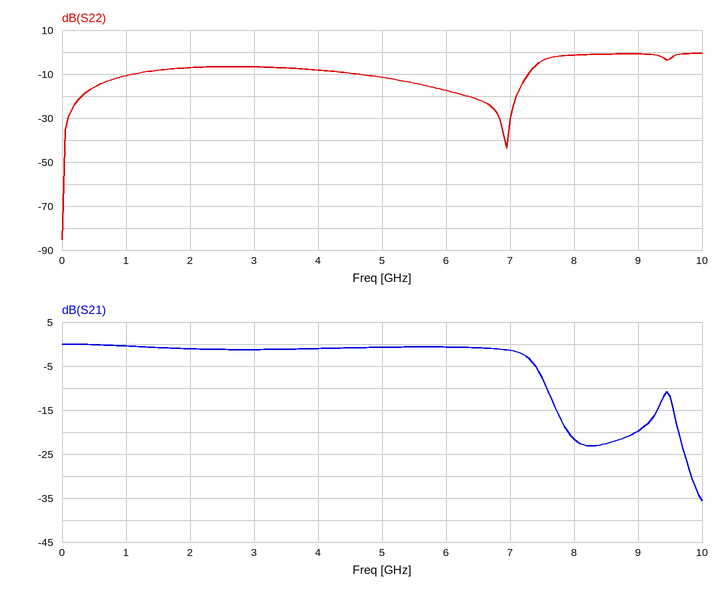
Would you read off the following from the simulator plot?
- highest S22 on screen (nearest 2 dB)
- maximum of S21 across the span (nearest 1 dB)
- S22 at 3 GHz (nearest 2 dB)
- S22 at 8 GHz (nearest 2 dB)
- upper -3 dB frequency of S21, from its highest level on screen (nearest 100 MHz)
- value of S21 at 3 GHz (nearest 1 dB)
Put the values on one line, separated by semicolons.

0 dB; 0 dB; -6 dB; -2 dB; 7.3 GHz; -1 dB
